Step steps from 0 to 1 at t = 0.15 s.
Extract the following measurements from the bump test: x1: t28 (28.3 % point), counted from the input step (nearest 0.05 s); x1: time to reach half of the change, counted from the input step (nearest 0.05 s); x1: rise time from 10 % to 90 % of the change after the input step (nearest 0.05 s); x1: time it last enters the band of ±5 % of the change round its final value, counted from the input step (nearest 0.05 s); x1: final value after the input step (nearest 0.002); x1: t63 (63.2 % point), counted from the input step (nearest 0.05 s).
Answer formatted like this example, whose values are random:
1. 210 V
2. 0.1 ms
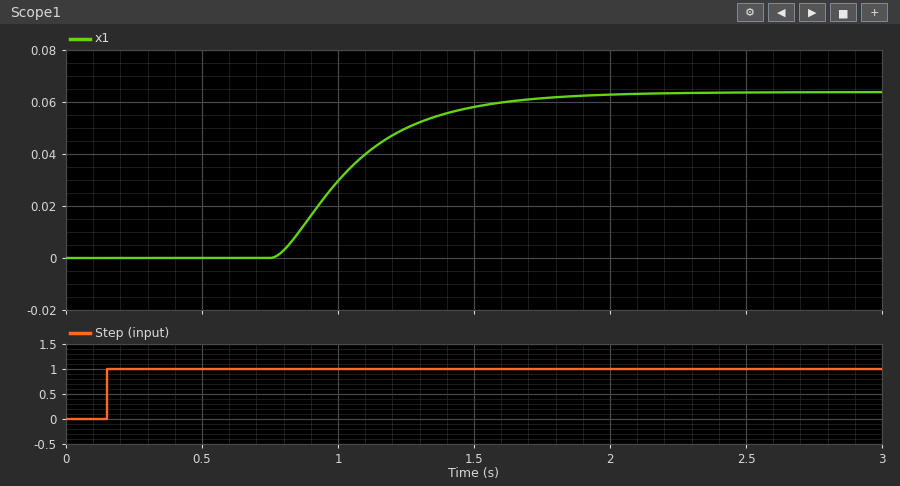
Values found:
1. 0.75 s
2. 0.85 s
3. 0.65 s
4. 1.50 s
5. 0.064
6. 0.95 s
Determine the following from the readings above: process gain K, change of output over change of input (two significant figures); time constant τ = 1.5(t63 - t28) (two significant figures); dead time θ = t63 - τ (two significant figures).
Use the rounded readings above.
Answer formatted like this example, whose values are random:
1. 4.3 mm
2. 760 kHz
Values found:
1. 0.064
2. 0.30 s
3. 0.65 s
